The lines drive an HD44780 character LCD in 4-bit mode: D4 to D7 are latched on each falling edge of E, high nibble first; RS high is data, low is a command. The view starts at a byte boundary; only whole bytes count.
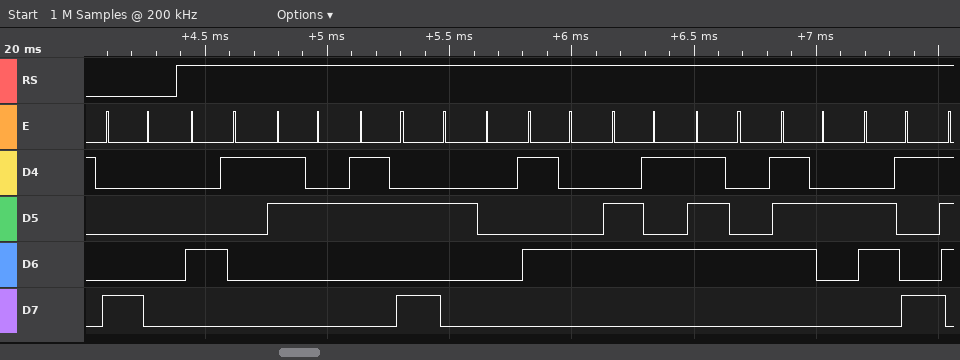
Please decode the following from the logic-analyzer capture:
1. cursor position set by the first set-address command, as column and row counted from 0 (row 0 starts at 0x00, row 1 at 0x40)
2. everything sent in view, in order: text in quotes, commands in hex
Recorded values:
column 0, row 0
0x80 "A2: Tetri"
